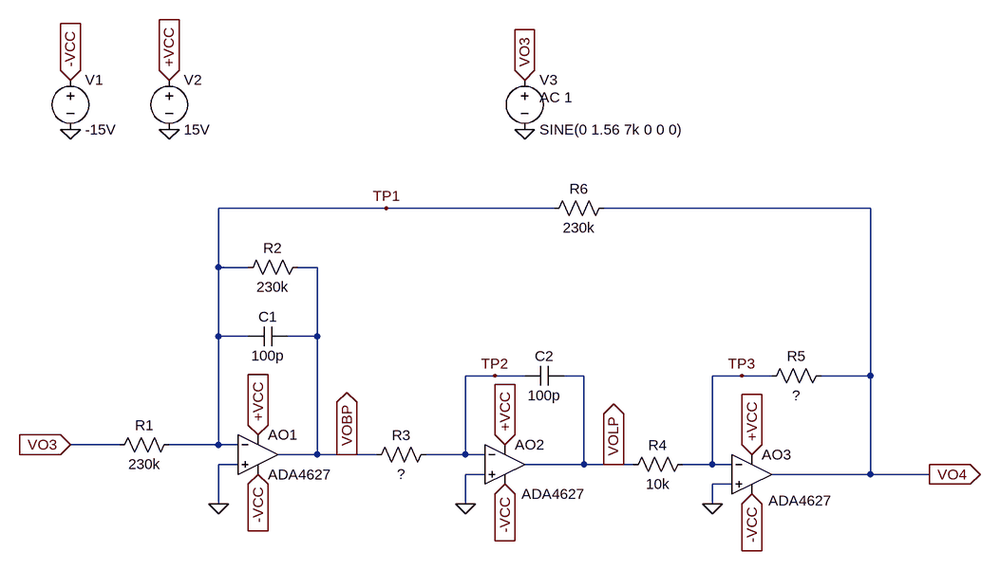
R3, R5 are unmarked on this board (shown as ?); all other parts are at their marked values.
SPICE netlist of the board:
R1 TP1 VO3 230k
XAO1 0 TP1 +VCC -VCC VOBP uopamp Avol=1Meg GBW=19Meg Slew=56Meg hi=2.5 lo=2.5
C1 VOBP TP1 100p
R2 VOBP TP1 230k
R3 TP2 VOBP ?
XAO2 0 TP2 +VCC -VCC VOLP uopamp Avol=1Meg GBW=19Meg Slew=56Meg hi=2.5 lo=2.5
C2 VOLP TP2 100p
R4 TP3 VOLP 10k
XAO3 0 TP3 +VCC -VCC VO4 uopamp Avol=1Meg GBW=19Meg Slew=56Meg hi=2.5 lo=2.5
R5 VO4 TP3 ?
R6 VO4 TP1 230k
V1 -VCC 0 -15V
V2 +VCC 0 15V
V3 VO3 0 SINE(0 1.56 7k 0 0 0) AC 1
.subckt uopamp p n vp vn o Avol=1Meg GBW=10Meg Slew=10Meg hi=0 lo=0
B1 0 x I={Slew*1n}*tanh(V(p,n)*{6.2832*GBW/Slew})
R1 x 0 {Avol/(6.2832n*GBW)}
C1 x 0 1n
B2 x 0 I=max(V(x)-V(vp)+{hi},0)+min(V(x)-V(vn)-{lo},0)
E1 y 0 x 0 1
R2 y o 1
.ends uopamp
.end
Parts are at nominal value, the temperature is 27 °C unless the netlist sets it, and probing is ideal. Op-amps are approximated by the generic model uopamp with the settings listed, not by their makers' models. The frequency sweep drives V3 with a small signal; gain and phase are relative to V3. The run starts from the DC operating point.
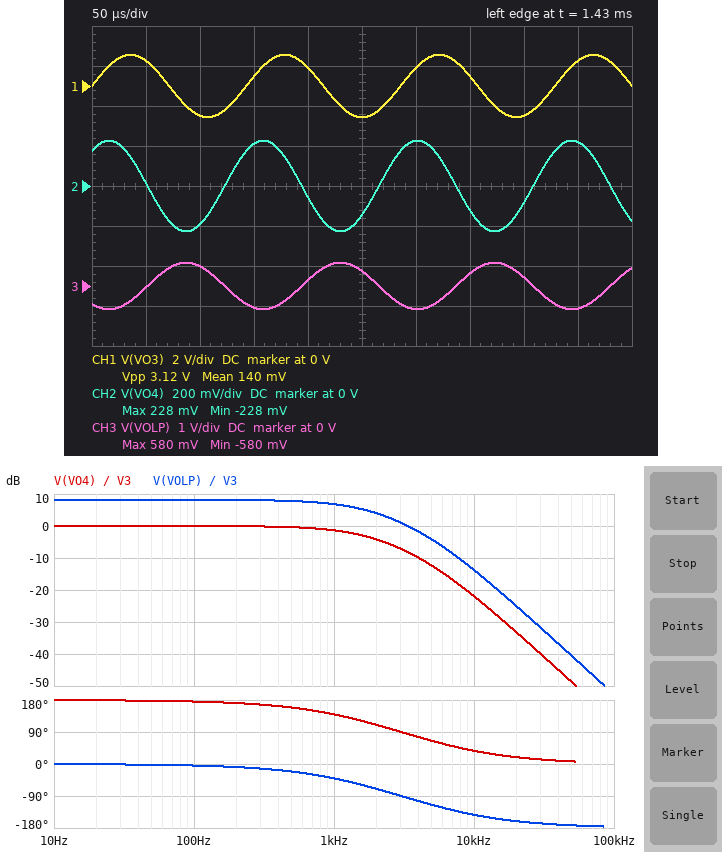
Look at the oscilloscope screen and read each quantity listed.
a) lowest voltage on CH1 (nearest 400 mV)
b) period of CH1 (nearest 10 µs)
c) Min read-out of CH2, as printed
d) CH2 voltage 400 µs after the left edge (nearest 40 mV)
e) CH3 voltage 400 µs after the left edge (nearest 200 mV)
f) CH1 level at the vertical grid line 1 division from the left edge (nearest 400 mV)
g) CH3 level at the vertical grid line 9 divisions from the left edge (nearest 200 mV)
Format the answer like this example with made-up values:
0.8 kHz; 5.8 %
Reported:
-1.6 V; 140 µs; -228 mV; -80 mV; 200 mV; 1.2 V; -600 mV
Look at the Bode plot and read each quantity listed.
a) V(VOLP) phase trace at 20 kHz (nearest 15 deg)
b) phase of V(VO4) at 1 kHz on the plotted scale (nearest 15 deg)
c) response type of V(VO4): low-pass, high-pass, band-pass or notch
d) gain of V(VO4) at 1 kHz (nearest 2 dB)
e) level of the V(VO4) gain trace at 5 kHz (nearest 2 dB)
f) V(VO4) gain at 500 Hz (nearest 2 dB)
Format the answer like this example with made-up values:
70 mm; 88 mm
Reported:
-165 deg; 135 deg; low-pass; -2 dB; -12 dB; 0 dB
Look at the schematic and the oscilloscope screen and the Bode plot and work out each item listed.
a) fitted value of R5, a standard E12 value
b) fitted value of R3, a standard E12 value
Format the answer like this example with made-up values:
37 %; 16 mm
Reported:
3.9 kΩ; 470 kΩ
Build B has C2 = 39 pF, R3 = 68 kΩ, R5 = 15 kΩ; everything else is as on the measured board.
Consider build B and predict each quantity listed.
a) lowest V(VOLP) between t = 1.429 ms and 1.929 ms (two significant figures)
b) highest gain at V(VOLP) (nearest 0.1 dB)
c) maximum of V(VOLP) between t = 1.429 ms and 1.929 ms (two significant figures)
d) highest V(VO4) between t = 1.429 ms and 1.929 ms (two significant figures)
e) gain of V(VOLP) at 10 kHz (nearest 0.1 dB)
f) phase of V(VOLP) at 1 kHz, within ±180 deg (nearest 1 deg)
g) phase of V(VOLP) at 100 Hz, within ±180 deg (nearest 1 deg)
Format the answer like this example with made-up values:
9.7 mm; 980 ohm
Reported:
-1.1 V; 7.9 dB; 1.1 V; 1.7 V; -2.1 dB; -1 deg; 0 deg
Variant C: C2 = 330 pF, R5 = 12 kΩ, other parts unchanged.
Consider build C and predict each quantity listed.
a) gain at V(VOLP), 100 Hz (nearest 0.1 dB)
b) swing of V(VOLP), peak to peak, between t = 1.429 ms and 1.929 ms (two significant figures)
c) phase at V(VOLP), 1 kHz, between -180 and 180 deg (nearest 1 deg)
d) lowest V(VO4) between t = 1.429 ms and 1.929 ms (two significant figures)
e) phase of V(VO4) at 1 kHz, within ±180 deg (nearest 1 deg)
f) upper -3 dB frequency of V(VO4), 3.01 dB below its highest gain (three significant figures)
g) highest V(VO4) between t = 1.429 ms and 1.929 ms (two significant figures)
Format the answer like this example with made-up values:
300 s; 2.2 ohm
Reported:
-1.6 dB; 350 mV; -43 deg; -210 mV; 137 deg; 1.48 kHz; 210 mV
